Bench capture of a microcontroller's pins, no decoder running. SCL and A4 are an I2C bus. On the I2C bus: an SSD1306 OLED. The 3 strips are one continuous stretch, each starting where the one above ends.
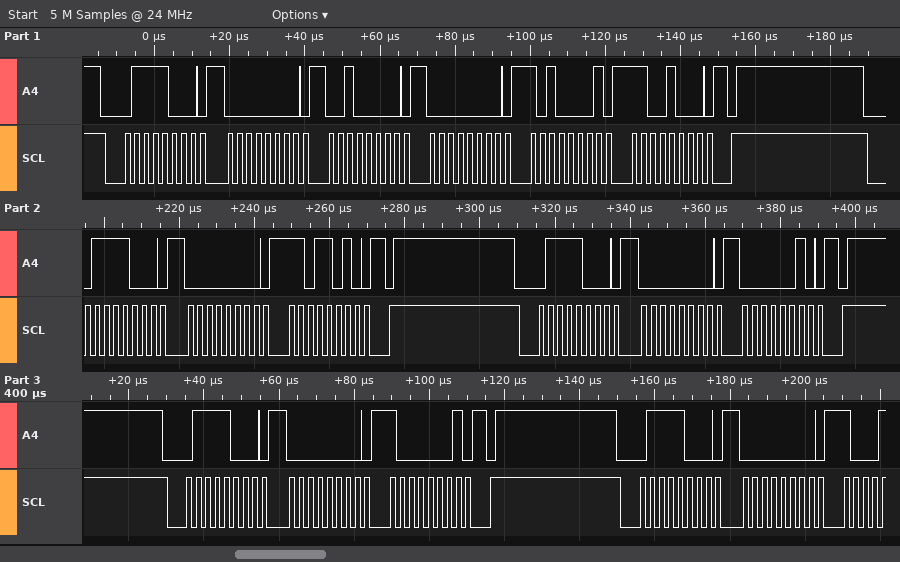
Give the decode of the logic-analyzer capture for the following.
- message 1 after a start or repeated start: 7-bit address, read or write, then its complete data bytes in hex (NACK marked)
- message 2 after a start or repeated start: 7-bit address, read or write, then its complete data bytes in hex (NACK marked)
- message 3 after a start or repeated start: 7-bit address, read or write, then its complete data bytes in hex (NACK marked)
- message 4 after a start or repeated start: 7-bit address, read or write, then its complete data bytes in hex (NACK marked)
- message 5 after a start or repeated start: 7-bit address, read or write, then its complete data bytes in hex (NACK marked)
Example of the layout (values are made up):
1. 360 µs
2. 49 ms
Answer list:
1. 0x3C write: 00 20 00 A1 C8
2. 0x3C write: 00 DA
3. 0x3C write: 00 02
4. 0x3C write: 00 81
5. 0x3C write: 00
